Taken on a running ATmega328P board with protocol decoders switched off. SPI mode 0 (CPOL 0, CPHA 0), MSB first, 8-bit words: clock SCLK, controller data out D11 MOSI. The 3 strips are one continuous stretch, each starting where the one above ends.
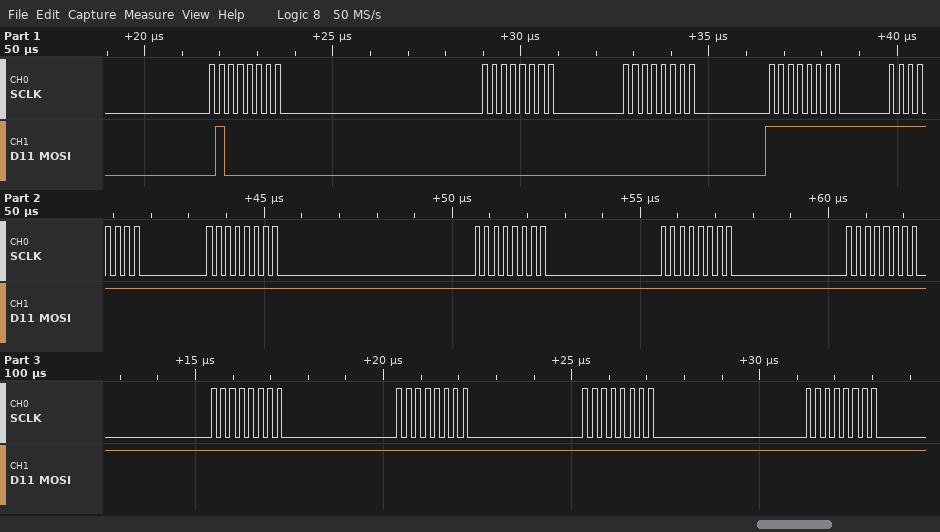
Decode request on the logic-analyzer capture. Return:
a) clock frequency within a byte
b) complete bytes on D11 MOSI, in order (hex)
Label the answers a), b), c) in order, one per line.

a) 4 MHz
b) 40 00 00 FF FF FF FF FF FF FF FF FF FF
